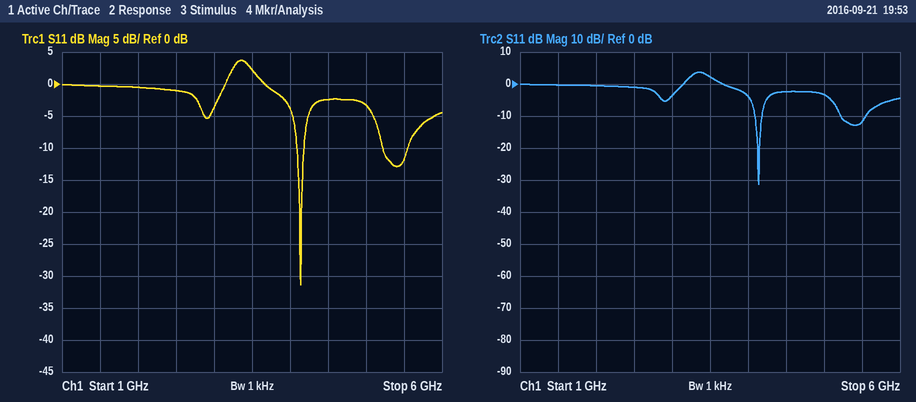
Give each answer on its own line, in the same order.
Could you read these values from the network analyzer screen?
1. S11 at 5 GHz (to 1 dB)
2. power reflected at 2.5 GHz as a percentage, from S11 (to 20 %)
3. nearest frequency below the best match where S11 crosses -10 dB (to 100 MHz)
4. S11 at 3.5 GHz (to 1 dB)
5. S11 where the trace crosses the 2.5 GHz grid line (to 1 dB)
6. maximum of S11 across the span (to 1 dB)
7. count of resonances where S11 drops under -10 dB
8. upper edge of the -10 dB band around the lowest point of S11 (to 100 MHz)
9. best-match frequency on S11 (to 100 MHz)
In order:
-3 dB
80 %
4.1 GHz
2 dB
-1 dB
4 dB
2
4.2 GHz
4.1 GHz
